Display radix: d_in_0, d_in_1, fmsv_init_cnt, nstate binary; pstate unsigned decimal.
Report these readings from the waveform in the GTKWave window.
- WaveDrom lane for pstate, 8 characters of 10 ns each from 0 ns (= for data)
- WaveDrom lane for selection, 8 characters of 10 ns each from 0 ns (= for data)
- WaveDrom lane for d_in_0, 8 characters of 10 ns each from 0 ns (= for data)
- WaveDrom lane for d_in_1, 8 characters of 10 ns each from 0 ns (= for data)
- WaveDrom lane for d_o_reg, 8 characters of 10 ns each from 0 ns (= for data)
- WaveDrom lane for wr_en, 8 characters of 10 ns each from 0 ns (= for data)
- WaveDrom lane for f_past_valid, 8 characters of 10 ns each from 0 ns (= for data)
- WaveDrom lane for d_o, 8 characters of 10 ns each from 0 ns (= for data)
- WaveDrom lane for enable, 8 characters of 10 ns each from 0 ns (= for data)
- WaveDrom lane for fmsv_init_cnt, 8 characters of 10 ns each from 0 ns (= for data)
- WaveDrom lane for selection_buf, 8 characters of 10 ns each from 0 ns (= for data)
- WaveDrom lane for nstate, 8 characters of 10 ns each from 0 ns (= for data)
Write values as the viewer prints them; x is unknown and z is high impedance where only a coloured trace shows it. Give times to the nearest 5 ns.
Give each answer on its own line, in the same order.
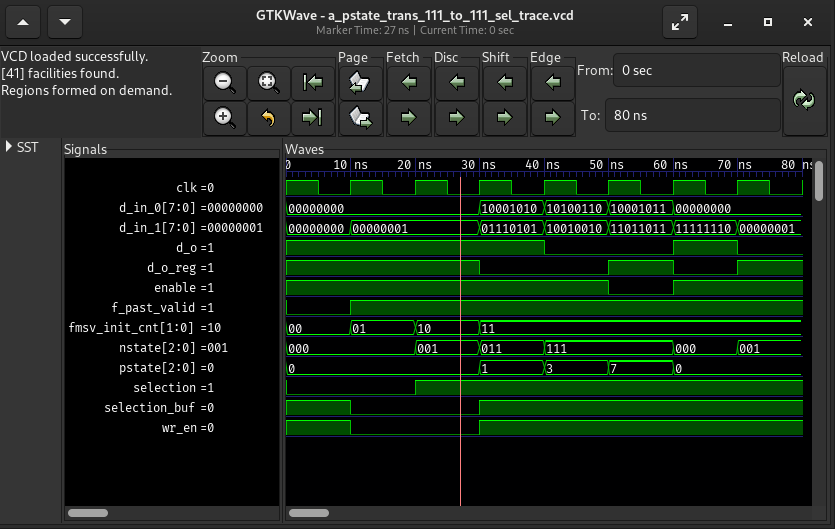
{name: 'pstate', wave: '=..====.', data: '0 1 3 7 0'}
{name: 'selection', wave: '0.1.....'}
{name: 'd_in_0', wave: '=..====.', data: '00000000 10001010 10100110 10001011 00000000'}
{name: 'd_in_1', wave: '==.=====', data: '00000000 00000001 01110101 10010010 11011011 11111110 00000001'}
{name: 'd_o_reg', wave: '1..0.101'}
{name: 'wr_en', wave: '10.1....'}
{name: 'f_past_valid', wave: '01......'}
{name: 'd_o', wave: '1...0.10'}
{name: 'enable', wave: '1....01.'}
{name: 'fmsv_init_cnt', wave: '====....', data: '00 01 10 11'}
{name: 'selection_buf', wave: '10.1....'}
{name: 'nstate', wave: '=.===.==', data: '000 001 011 111 000 001'}
